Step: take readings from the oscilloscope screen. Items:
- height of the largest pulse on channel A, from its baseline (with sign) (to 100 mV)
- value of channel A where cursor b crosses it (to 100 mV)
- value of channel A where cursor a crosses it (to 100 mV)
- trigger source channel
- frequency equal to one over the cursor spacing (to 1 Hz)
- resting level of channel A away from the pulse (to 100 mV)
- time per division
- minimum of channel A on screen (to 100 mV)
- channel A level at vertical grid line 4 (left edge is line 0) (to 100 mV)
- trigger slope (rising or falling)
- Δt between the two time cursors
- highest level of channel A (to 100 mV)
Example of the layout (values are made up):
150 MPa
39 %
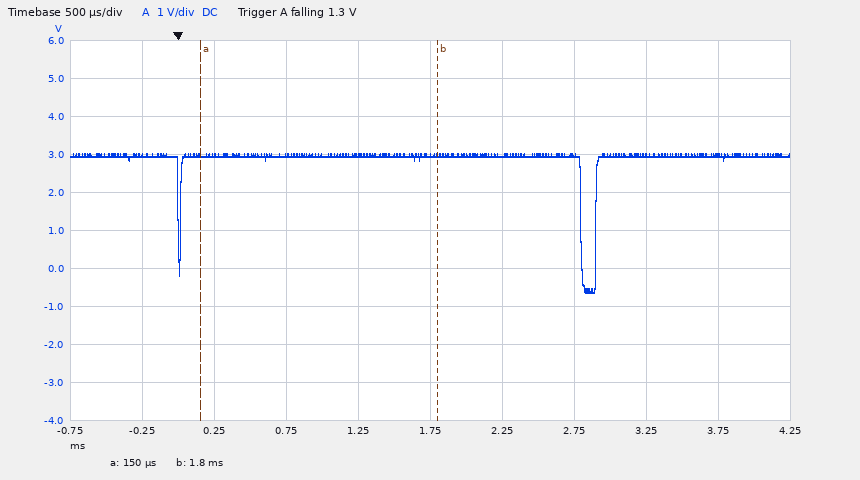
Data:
-3.6 V
3.0 V
3.0 V
channel A
606 Hz
3.0 V
500 µs
-600 mV
3.0 V
falling
1.65 ms
3.0 V
